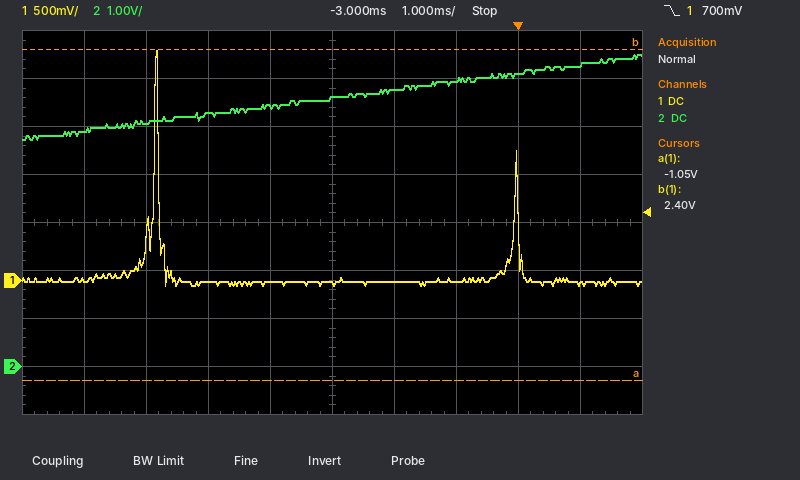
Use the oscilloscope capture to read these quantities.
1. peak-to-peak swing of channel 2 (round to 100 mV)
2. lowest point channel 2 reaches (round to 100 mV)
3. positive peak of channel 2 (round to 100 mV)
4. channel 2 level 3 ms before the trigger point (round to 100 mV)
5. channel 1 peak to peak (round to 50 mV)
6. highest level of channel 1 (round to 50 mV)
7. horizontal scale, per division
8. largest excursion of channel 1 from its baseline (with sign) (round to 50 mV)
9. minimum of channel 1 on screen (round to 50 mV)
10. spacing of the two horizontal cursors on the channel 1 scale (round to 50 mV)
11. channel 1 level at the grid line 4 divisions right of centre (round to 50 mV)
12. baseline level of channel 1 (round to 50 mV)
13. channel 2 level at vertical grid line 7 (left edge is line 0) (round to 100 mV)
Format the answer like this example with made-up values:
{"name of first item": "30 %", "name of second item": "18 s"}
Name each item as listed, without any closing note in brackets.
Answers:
{"peak-to-peak swing of channel 2": "1.8 V", "lowest point channel 2 reaches": "4.7 V", "positive peak of channel 2": "6.5 V", "channel 2 level 3 ms before the trigger point": "5.6 V", "channel 1 peak to peak": "2.45 V", "highest level of channel 1": "2.40 V", "horizontal scale, per division": "1 ms", "largest excursion of channel 1 from its baseline (with sign)": "+2.40 V", "minimum of channel 1 on screen": "-50 mV", "spacing of the two horizontal cursors on the channel 1 scale": "3.45 V", "channel 1 level at the grid line 4 divisions right of centre": "-50 mV", "baseline level of channel 1": "0 mV", "channel 2 level at vertical grid line 7 (left edge is line 0)": "6.0 V"}
